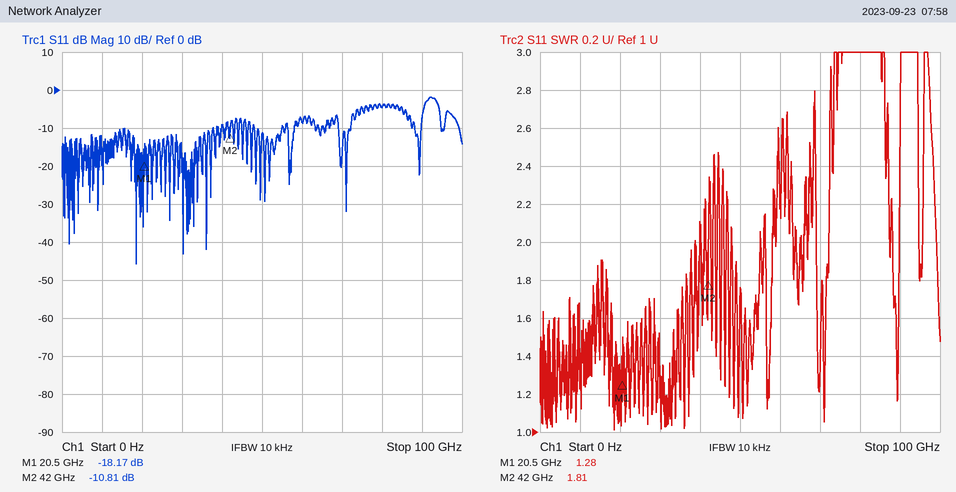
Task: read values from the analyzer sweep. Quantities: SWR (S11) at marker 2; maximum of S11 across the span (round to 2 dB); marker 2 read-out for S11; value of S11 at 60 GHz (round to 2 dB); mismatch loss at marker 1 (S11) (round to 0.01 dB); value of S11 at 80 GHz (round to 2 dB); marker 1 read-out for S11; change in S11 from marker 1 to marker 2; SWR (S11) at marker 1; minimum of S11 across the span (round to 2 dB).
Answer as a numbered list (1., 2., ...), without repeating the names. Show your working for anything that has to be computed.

1. 1.81
2. -2 dB
3. -10.81 dB
4. -8 dB
5. −10 log10(1 − 10^(-18.17/10)) ≈ 0.07 dB
6. -4 dB
7. -18.17 dB
8. -10.81 − (-18.17) = 7.36 dB
9. 1.28
10. -46 dB
